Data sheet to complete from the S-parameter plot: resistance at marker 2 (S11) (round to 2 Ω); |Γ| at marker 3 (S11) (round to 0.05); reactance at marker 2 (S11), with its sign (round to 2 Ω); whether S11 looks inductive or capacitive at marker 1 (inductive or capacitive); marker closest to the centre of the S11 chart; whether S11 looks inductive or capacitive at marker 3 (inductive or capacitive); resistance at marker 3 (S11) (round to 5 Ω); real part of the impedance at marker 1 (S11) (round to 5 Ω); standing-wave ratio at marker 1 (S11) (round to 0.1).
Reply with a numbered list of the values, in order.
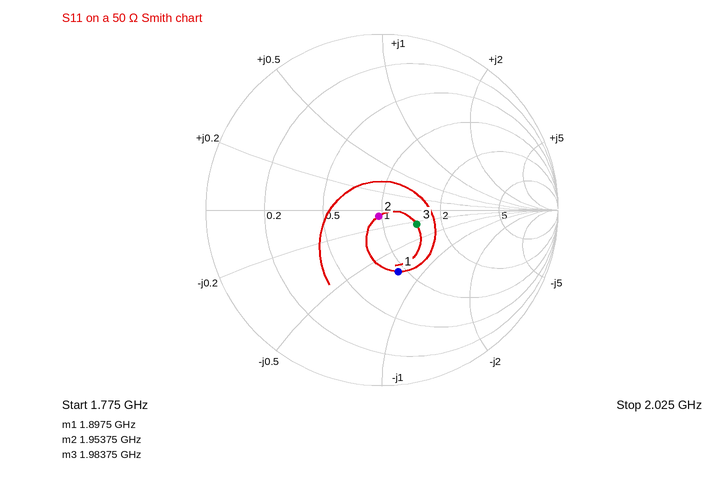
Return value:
1. 48 Ω
2. 0.20
3. -4 Ω
4. capacitive
5. marker 2
6. capacitive
7. 75 Ω
8. 45 Ω
9. 2.1
